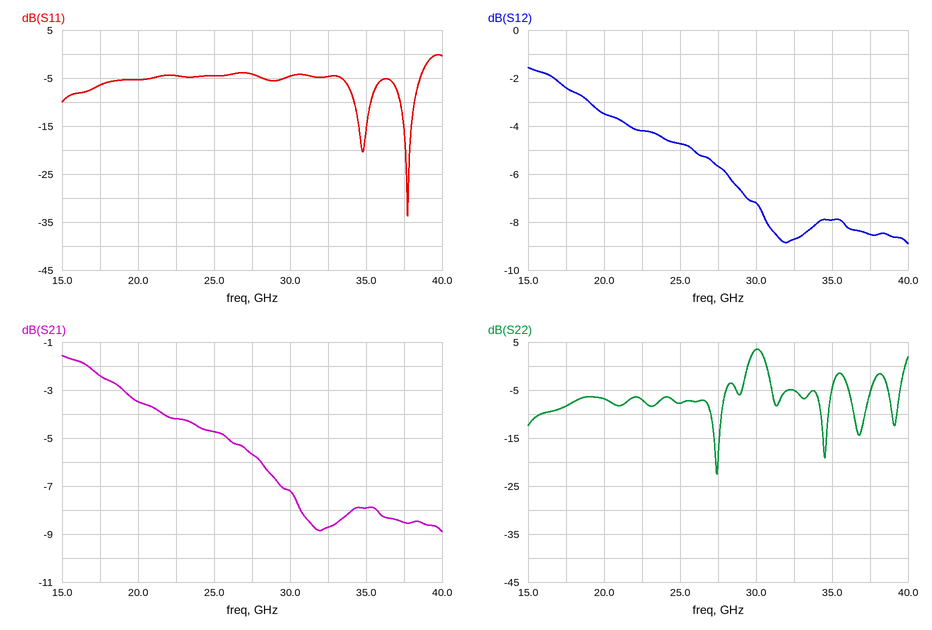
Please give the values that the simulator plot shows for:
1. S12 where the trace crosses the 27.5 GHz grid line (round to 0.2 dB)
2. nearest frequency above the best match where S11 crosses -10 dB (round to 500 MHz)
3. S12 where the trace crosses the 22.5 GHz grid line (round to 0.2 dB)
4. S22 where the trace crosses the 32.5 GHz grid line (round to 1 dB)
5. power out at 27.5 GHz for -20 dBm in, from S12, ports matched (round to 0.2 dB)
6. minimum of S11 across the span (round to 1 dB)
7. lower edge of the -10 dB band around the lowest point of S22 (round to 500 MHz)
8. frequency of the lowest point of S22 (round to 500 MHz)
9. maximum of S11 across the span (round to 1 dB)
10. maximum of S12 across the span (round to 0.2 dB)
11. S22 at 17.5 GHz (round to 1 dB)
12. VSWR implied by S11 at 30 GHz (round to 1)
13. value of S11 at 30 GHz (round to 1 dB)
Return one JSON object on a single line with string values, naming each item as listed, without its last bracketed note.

{"S12 where the trace crosses the 27.5 GHz grid line": "-5.6 dB", "nearest frequency above the best match where S11 crosses -10 dB": "38.0 GHz", "S12 where the trace crosses the 22.5 GHz grid line": "-4.2 dB", "S22 where the trace crosses the 32.5 GHz grid line": "-5 dB", "power out at 27.5 GHz for -20 dBm in, from S12, ports matched": "-25.6 dBm", "minimum of S11 across the span": "-34 dB", "lower edge of the -10 dB band around the lowest point of S22": "27.0 GHz", "frequency of the lowest point of S22": "27.5 GHz", "maximum of S11 across the span": "0 dB", "maximum of S12 across the span": "-1.6 dB", "S22 at 17.5 GHz": "-8 dB", "VSWR implied by S11 at 30 GHz": "4", "value of S11 at 30 GHz": "-5 dB"}
